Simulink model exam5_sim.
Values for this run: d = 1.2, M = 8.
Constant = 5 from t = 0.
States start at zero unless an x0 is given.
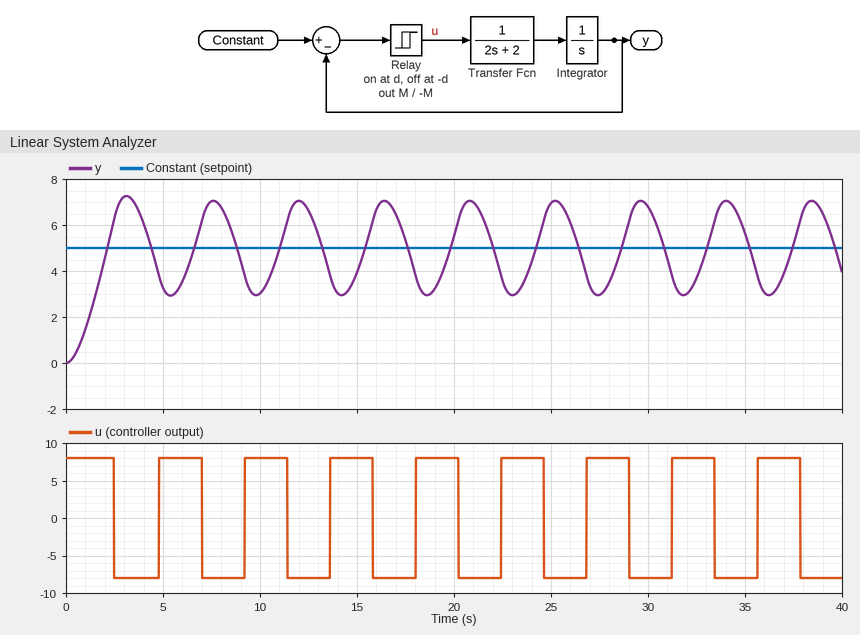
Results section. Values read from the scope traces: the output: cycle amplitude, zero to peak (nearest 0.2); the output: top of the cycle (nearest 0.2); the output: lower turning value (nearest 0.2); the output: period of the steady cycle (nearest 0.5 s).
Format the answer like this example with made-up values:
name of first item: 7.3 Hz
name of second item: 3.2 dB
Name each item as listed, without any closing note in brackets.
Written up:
the output: cycle amplitude, zero to peak: 2.0
the output: top of the cycle: 7.0
the output: lower turning value: 3.0
the output: period of the steady cycle: 4.5 s
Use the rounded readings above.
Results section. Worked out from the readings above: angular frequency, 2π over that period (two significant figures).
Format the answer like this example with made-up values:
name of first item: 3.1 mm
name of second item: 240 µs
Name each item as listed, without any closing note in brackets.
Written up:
angular frequency, 2π over that period: 1.4 rad/s
